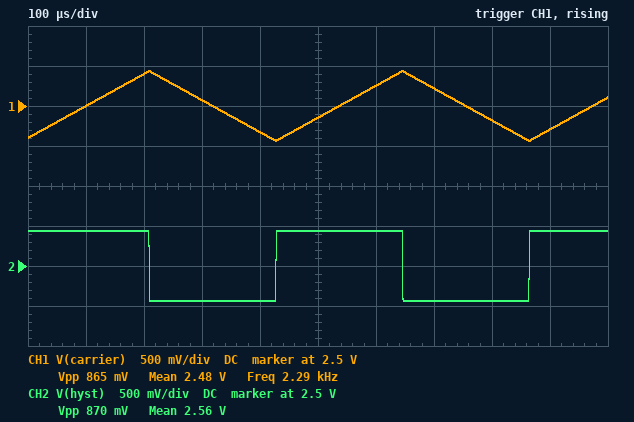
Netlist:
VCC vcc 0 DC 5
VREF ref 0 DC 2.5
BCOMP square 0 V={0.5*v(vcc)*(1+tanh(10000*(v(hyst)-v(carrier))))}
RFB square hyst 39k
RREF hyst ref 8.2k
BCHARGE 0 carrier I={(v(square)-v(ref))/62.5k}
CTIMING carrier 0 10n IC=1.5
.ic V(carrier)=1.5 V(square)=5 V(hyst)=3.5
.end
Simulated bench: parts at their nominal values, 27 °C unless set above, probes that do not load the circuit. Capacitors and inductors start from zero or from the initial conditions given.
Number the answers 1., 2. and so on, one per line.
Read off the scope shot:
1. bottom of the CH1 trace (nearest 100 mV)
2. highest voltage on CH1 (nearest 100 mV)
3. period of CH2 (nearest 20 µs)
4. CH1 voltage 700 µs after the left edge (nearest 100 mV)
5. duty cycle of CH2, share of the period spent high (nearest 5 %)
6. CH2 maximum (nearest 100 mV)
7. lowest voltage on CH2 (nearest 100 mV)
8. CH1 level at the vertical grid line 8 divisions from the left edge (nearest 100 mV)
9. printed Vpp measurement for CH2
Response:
1. 2.1 V
2. 2.9 V
3. 440 µs
4. 2.7 V
5. 50 %
6. 2.9 V
7. 2.1 V
8. 2.3 V
9. 870 mV
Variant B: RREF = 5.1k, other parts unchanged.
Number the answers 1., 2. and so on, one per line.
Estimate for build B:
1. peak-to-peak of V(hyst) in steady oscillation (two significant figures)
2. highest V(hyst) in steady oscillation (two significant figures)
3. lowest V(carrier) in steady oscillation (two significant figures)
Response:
1. 580 mV
2. 2.8 V
3. 2.2 V
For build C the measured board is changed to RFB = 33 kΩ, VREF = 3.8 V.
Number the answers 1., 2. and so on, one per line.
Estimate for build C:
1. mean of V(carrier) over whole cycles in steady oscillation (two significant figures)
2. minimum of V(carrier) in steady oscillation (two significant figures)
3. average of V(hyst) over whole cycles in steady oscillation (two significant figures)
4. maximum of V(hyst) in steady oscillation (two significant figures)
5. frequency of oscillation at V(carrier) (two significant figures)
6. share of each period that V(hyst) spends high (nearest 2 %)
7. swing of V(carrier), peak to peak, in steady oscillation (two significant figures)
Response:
1. 3.5 V
2. 3.0 V
3. 3.8 V
4. 4.0 V
5. 1.5 kHz
6. 76 %
7. 990 mV
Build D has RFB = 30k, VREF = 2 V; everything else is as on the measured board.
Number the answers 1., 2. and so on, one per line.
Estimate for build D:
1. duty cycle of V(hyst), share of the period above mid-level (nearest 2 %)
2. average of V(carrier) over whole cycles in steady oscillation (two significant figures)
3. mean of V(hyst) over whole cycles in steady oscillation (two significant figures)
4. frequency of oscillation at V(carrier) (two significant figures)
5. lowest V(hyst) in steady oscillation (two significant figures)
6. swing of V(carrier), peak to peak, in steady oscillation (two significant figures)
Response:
1. 40 %
2. 2.1 V
3. 2.0 V
4. 1.8 kHz
5. 1.6 V
6. 1.1 V
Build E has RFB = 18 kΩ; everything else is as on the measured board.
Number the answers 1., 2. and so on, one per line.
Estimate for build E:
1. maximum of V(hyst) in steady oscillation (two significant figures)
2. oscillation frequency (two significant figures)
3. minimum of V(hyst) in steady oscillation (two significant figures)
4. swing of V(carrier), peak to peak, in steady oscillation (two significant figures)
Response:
1. 3.3 V
2. 1.3 kHz
3. 1.7 V
4. 1.6 V
